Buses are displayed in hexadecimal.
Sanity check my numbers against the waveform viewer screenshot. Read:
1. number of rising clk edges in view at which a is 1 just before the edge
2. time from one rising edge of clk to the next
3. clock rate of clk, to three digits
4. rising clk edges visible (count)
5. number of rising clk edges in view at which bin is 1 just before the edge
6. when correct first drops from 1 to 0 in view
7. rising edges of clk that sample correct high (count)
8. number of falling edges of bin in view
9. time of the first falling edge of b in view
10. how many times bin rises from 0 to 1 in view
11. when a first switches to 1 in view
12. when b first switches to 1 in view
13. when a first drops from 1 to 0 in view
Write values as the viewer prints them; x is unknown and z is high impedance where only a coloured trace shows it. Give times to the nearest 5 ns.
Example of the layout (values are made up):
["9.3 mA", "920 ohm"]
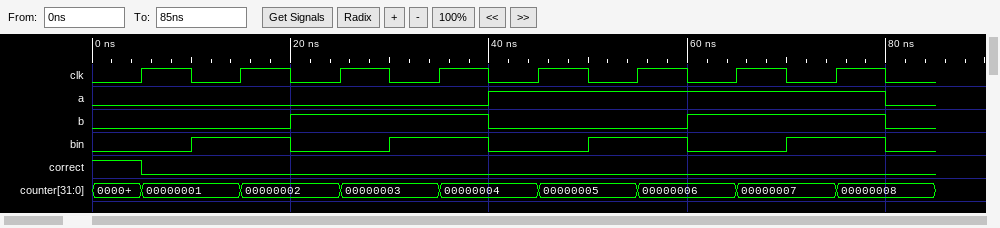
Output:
["4", "10 ns", "100 MHz", "8", "4", "5 ns", "1", "4", "40 ns", "4", "40 ns", "20 ns", "80 ns"]
